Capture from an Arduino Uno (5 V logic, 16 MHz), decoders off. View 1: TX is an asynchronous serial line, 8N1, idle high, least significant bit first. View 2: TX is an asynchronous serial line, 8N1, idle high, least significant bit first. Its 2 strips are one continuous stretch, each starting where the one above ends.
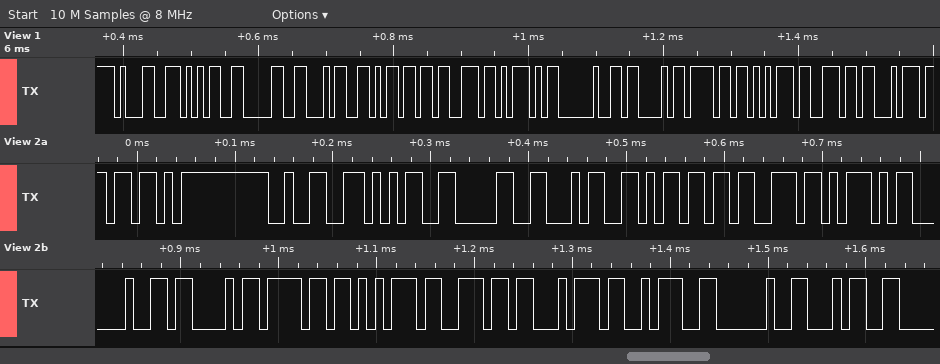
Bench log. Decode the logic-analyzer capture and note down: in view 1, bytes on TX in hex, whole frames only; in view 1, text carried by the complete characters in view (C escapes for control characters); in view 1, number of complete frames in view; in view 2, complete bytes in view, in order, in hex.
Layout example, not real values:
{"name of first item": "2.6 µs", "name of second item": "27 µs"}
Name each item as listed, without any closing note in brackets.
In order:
{"in view 1, bytes on TX in hex, whole frames only": "31 35 30 34 6D 73 5D 20 43 6F 75 6E 74", "in view 1, text carried by the complete characters in view": "\"1504ms] Count\"", "in view 1, number of complete frames in view": "13", "in view 2, complete bytes in view, in order, in hex": "5B 32 35 30 34 6D 73 5D 20 43 6F 75 6E 74 3A 20 34"}
